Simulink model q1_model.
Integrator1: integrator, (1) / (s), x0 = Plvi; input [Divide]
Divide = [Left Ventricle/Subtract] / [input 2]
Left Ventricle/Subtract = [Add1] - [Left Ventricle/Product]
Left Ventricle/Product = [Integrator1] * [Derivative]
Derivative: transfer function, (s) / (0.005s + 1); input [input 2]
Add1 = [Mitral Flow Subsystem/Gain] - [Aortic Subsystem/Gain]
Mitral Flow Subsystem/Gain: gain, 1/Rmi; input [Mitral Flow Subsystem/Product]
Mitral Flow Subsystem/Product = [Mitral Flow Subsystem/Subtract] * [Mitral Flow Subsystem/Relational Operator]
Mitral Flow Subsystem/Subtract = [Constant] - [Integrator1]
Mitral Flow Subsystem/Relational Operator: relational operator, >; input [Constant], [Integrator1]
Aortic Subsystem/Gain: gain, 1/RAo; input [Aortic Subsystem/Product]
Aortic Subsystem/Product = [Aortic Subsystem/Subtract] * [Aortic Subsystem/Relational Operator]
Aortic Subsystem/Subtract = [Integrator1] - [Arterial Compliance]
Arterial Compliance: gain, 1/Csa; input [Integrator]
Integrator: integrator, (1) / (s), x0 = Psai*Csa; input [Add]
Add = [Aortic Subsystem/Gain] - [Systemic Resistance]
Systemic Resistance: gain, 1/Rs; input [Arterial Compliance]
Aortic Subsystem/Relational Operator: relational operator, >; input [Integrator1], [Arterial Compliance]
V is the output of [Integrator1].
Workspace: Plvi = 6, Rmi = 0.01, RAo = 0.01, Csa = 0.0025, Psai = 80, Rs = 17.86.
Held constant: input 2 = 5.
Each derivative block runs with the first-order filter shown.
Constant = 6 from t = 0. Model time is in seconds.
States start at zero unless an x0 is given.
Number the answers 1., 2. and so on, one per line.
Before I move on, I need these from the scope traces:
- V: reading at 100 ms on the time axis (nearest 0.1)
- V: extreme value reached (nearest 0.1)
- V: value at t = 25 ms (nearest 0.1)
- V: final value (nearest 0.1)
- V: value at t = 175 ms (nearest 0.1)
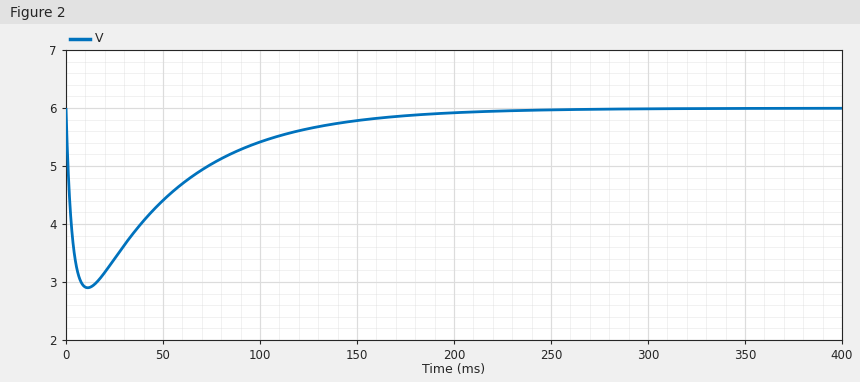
1. 5.4
2. 2.9
3. 3.4
4. 6.0
5. 5.9
